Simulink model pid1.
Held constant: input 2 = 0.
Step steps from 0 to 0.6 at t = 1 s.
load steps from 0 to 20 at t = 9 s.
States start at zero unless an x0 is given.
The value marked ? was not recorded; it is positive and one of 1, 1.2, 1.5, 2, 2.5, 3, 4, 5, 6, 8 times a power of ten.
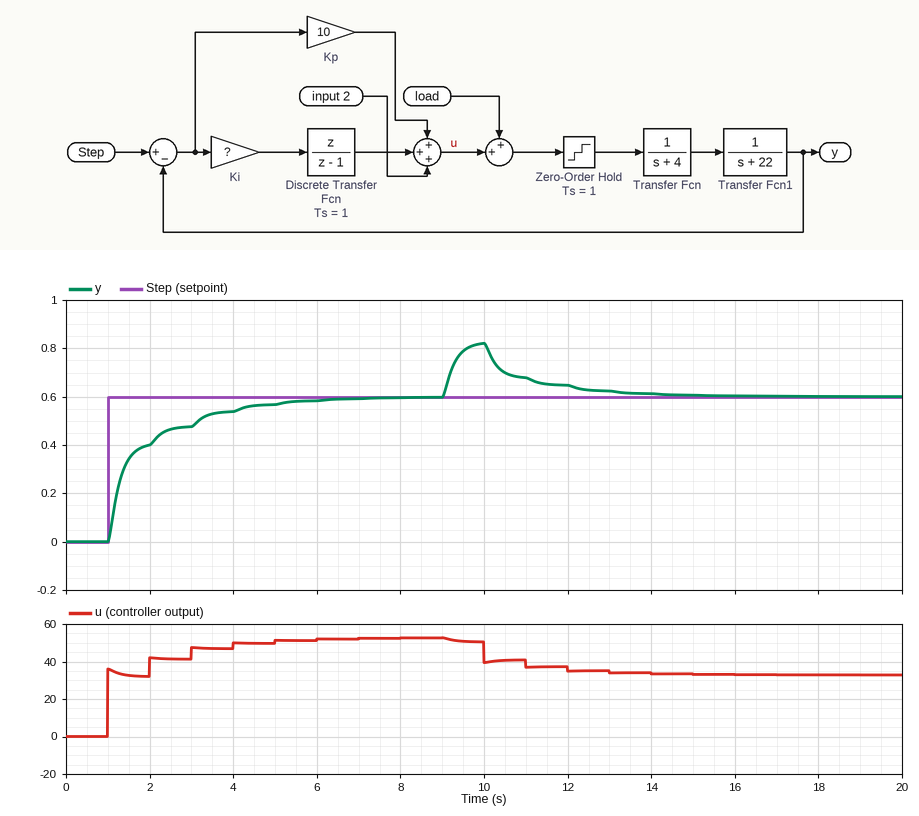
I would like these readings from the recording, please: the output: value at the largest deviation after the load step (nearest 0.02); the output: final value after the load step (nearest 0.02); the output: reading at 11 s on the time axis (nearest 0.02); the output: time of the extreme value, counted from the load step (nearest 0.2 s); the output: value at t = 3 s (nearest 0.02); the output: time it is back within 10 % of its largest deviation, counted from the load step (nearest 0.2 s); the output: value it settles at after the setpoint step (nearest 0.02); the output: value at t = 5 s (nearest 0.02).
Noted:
0.82
0.60
0.68
1.0 s
0.48
4.0 s
0.60
0.56
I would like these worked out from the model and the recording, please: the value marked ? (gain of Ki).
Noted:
50
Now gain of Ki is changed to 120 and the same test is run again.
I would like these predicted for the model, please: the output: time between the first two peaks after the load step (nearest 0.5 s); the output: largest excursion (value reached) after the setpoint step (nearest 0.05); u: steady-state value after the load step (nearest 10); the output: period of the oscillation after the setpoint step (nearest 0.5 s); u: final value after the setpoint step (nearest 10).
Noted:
2.0 s
0.85
30
2.0 s
50
